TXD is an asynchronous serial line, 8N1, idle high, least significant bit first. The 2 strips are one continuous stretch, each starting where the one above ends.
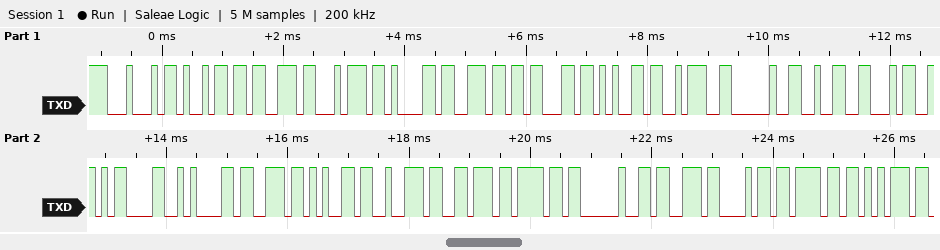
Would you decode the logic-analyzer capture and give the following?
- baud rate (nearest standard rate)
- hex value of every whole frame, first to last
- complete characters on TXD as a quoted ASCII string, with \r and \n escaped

9600 baud
44 69 73 74 61 6E 63 65 3A 20 32 34 0D 0A 73 65 72 76 6F 20 73 68 6F 75
"Distance: 24\r\nservo shou"
